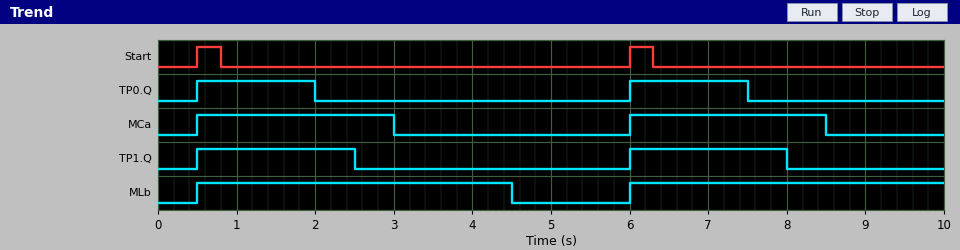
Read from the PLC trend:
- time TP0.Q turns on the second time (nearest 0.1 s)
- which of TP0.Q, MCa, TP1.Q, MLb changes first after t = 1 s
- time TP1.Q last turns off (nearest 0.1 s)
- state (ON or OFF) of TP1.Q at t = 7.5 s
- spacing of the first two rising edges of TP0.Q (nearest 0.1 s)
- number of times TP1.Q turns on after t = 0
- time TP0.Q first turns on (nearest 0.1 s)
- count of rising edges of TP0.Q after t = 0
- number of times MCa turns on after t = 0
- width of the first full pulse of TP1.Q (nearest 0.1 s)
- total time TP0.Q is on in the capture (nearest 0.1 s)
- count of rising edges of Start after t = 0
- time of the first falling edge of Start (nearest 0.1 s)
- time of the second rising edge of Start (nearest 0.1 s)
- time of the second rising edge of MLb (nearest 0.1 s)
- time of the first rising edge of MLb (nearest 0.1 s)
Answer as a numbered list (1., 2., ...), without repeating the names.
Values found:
1. 6.0 s
2. TP0.Q
3. 8.0 s
4. ON
5. 5.5 s
6. 2
7. 0.5 s
8. 2
9. 2
10. 2.0 s
11. 3.0 s
12. 2
13. 0.8 s
14. 6.0 s
15. 6.0 s
16. 0.5 s
